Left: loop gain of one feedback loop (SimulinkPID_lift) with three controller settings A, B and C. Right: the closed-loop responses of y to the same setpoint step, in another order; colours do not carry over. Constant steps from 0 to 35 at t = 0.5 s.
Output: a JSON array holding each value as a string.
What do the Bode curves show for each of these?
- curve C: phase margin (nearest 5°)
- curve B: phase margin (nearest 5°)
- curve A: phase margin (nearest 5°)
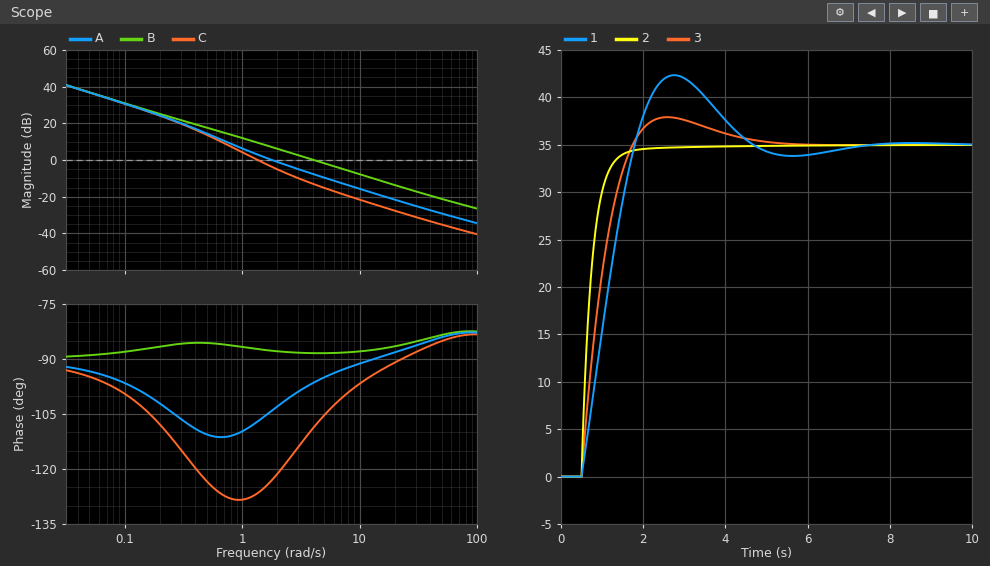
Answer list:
["55°", "90°", "75°"]
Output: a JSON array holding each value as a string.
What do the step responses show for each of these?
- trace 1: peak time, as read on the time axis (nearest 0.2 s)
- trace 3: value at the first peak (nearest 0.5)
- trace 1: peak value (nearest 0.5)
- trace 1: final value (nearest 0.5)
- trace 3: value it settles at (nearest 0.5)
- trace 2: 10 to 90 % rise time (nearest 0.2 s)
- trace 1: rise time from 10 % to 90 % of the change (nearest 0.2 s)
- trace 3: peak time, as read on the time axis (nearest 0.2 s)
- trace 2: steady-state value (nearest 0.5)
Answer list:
["2.8 s", "38.0", "42.5", "35.0", "35.0", "0.6 s", "1.0 s", "2.6 s", "35.0"]
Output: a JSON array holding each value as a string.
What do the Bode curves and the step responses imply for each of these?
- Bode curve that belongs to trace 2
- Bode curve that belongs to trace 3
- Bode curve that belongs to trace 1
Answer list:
["B", "A", "C"]
